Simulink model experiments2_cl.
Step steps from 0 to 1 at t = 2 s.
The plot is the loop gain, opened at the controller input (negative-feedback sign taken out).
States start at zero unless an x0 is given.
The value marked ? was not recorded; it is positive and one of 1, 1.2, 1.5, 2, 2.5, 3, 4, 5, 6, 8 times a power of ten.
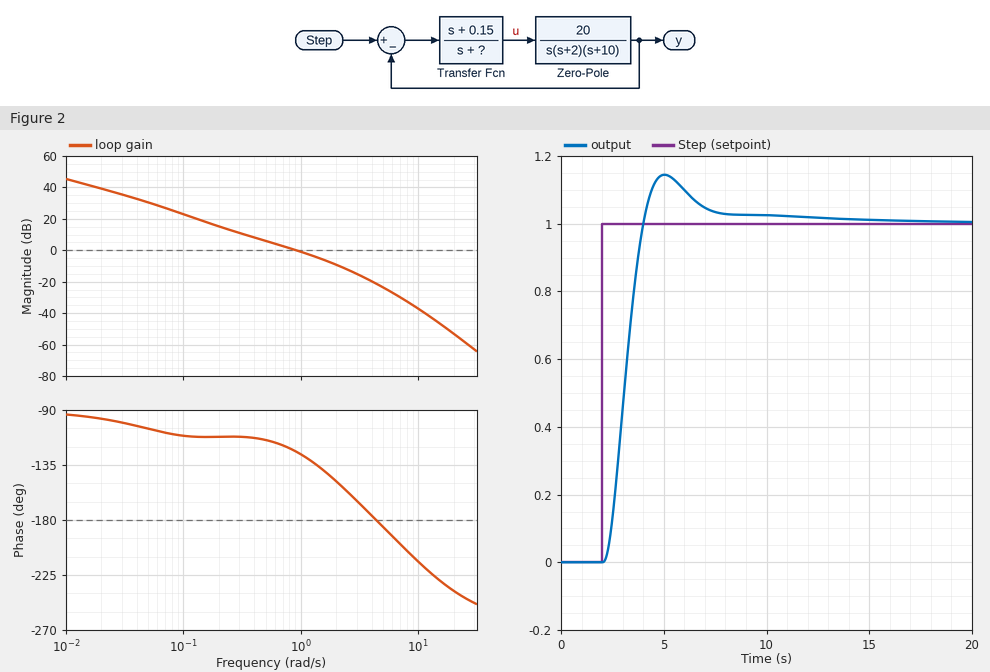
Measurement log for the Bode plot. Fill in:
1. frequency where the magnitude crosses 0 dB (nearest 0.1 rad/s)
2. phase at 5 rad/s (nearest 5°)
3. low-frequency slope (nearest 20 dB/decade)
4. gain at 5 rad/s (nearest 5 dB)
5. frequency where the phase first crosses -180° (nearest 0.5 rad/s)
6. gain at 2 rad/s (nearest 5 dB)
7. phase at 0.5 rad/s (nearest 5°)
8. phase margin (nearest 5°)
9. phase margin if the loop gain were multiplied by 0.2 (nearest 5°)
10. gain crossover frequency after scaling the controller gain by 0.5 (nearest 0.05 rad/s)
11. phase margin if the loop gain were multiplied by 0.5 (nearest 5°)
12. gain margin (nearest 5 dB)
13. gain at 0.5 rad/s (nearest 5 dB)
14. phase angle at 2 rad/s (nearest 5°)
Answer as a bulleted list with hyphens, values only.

- 0.9 rad/s
- -185°
- -20 dB/decade
- -25 dB
- 4.5 rad/s
- -10 dB
- -115°
- 55°
- 70°
- 0.50 rad/s
- 65°
- 20 dB
- 5 dB
- -150°
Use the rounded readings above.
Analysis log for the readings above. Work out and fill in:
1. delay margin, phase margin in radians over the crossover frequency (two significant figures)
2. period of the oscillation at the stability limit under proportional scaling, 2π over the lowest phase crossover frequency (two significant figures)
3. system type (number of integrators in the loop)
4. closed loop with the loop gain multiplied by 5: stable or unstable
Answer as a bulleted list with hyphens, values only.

- 1.1 s
- 1.4 s
- 1
- stable
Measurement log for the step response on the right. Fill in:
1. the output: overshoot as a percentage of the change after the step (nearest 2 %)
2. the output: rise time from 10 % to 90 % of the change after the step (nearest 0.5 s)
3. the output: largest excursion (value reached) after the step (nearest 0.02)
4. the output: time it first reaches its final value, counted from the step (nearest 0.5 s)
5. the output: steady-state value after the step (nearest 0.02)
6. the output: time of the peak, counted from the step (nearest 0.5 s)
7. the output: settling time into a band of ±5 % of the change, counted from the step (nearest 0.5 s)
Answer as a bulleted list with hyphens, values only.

- 14 %
- 1.5 s
- 1.14
- 2.0 s
- 1.00
- 3.0 s
- 5.0 s
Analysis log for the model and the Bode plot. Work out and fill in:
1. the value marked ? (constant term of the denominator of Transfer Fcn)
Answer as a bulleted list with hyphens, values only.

- 0.08
